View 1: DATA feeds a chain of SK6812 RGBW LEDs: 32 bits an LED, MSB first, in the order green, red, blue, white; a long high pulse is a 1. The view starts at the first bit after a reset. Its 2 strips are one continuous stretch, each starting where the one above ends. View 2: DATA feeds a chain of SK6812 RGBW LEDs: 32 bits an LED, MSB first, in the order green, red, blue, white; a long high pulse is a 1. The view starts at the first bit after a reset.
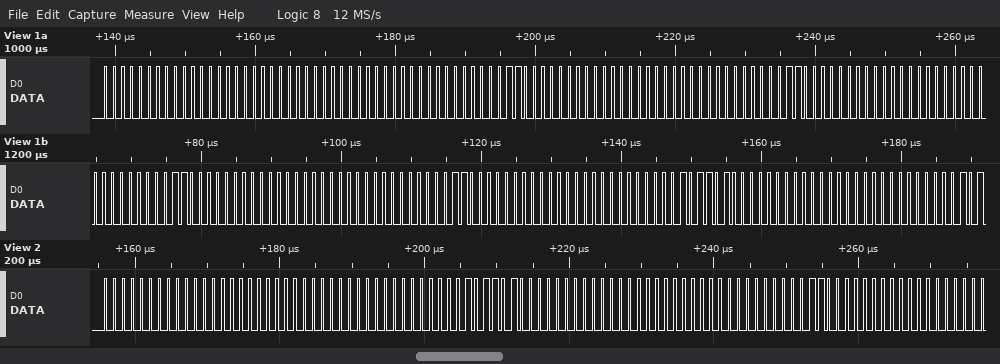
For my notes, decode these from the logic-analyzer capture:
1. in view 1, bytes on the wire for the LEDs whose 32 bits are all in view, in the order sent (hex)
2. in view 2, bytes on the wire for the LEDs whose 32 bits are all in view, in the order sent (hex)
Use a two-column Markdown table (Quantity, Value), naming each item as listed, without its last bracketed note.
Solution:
| Quantity | Value |
|---|---|
| in view 1, bytes on the wire for the LEDs whose 32 bits are all in view, in the order sent | 00 00 00 00 00 03 00 00 00 03 00 00 00 03 00 00 00 03 00 00 00 B4 00 00 |
| in view 2, bytes on the wire for the LEDs whose 32 bits are all in view, in the order sent | 00 00 00 00 00 B4 00 00 00 03 00 00 |
